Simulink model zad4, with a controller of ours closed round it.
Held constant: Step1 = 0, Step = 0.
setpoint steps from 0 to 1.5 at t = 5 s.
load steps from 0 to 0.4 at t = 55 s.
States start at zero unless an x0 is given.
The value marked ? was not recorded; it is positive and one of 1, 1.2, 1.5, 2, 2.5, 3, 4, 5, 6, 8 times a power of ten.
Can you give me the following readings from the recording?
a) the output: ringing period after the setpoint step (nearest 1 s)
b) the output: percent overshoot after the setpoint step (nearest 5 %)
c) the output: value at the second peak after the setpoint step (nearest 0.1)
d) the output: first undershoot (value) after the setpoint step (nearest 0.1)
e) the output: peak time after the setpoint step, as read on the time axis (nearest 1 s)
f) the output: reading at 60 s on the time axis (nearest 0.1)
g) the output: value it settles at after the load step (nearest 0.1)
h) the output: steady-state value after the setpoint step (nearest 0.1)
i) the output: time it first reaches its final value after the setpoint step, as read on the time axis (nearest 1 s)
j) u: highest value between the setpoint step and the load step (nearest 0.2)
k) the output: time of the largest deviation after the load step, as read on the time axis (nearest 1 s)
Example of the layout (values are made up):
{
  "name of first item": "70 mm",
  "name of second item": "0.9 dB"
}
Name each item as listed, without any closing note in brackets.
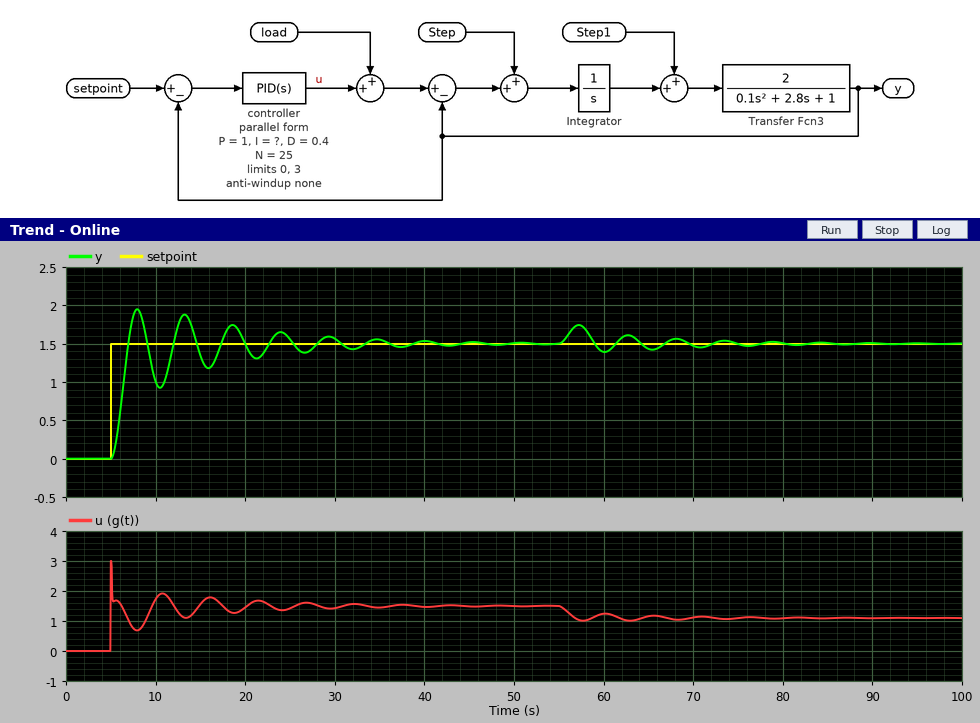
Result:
{
  "the output: ringing period after the setpoint step": "5 s",
  "the output: percent overshoot after the setpoint step": "30 %",
  "the output: value at the second peak after the setpoint step": "1.9",
  "the output: first undershoot (value) after the setpoint step": "0.9",
  "the output: peak time after the setpoint step, as read on the time axis": "8 s",
  "the output: reading at 60 s on the time axis": "1.4",
  "the output: value it settles at after the load step": "1.5",
  "the output: steady-state value after the setpoint step": "1.5",
  "the output: time it first reaches its final value after the setpoint step, as read on the time axis": "7 s",
  "u: highest value between the setpoint step and the load step": "3.0",
  "the output: time of the largest deviation after the load step, as read on the time axis": "57 s"
}
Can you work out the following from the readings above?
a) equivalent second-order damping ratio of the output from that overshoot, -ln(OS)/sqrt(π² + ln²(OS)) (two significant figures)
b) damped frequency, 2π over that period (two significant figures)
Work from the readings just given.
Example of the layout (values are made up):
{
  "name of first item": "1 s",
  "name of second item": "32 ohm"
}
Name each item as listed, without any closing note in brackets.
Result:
{
  "equivalent second-order damping ratio of the output from that overshoot, -ln(OS)/sqrt(π² + ln²(OS))": "0.36",
  "damped frequency, 2π over that period": "1.3 rad/s"
}
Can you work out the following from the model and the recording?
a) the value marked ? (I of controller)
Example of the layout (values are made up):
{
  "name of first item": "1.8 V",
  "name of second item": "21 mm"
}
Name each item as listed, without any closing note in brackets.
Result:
{
  "the value marked ?": "0.8"
}
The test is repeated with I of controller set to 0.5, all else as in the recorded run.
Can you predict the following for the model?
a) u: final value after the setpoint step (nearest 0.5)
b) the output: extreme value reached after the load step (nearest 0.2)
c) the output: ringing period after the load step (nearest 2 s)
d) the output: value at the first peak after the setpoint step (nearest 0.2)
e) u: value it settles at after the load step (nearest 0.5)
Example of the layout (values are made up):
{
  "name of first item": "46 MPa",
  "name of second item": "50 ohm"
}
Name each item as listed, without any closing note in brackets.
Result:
{
  "u: final value after the setpoint step": "1.5",
  "the output: extreme value reached after the load step": "1.8",
  "the output: ringing period after the load step": "6 s",
  "the output: value at the first peak after the setpoint step": "1.6",
  "u: value it settles at after the load step": "1.0"
}
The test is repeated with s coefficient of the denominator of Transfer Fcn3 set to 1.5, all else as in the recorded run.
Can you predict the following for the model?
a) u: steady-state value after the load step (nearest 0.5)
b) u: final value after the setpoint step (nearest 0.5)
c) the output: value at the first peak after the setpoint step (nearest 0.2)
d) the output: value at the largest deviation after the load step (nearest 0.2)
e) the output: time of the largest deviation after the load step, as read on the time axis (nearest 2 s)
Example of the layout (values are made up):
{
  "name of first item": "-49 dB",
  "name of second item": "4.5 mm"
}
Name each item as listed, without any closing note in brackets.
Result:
{
  "u: steady-state value after the load step": "1.0",
  "u: final value after the setpoint step": "1.5",
  "the output: value at the first peak after the setpoint step": "1.6",
  "the output: value at the largest deviation after the load step": "1.8",
  "the output: time of the largest deviation after the load step, as read on the time axis": "56 s"
}
